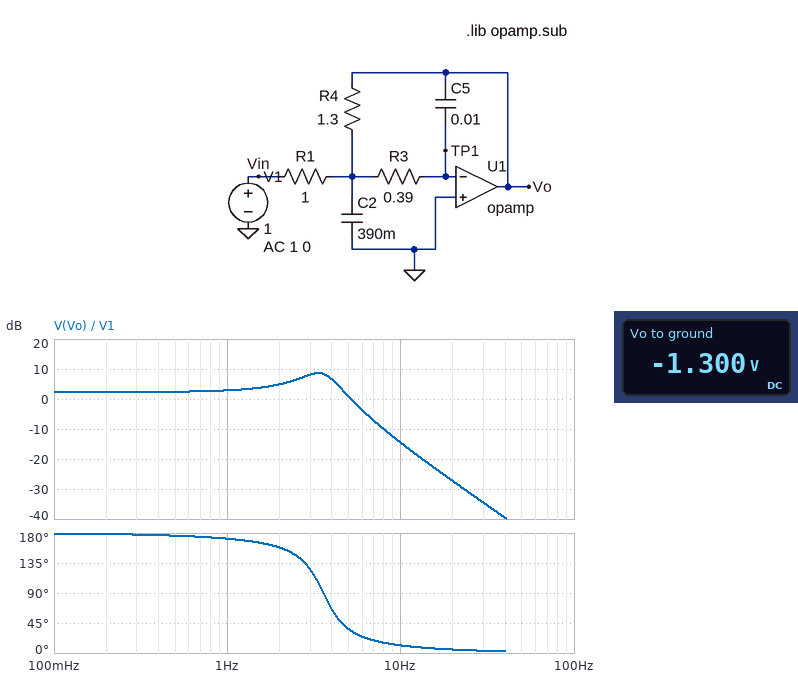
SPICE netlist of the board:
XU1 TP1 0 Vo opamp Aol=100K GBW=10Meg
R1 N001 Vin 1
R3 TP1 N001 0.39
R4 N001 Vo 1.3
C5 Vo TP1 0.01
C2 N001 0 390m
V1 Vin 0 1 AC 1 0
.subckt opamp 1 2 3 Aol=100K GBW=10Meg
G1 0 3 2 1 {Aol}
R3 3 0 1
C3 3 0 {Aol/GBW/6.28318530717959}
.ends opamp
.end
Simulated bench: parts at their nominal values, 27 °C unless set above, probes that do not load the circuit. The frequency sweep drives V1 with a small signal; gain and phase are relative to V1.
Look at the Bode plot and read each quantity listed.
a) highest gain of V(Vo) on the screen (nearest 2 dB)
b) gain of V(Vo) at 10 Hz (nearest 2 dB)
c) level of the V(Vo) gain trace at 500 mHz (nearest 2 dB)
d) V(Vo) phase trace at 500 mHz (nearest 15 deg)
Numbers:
8 dB
-14 dB
2 dB
180 deg
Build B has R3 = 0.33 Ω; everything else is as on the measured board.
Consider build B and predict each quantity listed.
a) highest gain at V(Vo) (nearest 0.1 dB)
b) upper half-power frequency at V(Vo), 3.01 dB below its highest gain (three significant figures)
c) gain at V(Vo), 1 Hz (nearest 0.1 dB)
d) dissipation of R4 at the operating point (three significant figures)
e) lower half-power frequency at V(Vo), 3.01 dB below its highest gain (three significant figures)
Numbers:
8.5 dB
4.54 Hz
2.8 dB
1.30 W
2.42 Hz
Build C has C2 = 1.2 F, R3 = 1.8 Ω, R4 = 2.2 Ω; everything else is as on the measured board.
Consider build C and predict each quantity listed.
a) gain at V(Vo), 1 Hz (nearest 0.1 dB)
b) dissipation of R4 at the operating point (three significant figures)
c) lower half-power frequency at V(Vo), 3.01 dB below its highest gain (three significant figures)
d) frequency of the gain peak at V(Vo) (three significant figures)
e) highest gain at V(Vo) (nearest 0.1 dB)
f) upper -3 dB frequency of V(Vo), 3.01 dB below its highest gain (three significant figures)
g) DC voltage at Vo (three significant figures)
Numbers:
6.8 dB
2.20 W
553 mHz
705 mHz
15.7 dB
830 mHz
-2.20 V
